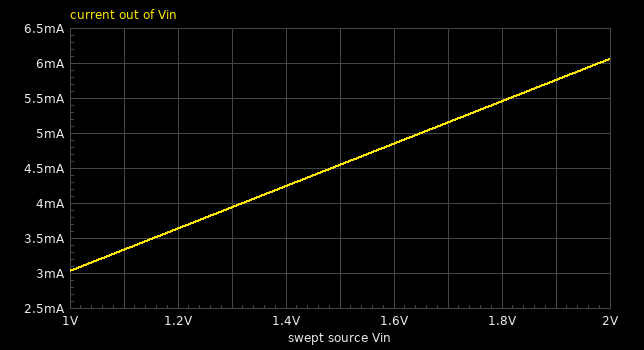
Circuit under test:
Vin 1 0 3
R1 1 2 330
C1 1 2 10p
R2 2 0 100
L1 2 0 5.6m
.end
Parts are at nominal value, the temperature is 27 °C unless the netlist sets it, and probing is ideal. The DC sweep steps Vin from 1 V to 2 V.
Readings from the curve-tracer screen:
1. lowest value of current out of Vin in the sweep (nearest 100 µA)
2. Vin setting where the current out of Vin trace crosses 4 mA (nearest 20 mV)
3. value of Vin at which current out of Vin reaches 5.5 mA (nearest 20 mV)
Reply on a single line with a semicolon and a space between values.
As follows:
3.0 mA; 1.32 V; 1.82 V
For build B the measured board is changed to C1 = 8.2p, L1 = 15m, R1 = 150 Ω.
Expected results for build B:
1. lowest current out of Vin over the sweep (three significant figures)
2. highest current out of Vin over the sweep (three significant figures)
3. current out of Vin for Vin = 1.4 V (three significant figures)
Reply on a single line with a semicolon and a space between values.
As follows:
6.67 mA; 13.3 mA; 9.33 mA
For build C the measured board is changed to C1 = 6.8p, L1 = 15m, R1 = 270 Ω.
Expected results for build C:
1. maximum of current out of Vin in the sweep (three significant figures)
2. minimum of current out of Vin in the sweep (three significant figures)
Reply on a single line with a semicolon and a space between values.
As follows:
7.41 mA; 3.70 mA
